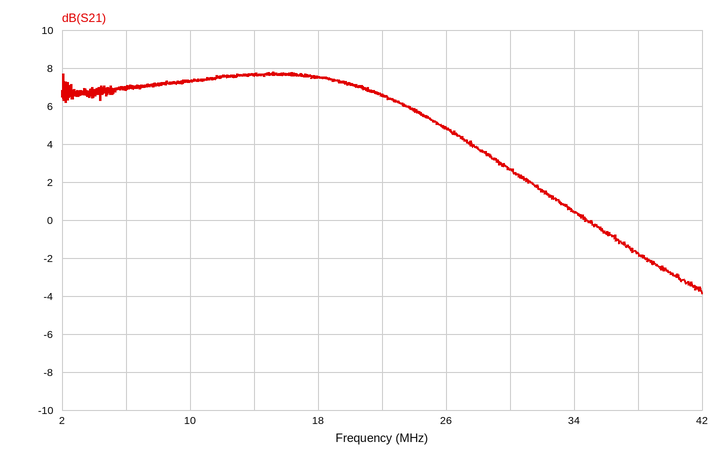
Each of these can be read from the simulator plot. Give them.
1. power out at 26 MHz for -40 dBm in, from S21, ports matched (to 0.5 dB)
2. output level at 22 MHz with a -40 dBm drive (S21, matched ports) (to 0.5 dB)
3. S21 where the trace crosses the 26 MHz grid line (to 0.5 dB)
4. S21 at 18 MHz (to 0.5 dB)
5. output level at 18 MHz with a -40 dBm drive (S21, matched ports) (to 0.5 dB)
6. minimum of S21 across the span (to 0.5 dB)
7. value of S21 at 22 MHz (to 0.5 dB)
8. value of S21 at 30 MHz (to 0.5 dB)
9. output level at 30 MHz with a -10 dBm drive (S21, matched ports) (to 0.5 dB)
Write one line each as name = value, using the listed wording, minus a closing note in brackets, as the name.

power out at 26 MHz for -40 dBm in, from S21, ports matched = -35.0 dBm
output level at 22 MHz with a -40 dBm drive (S21, matched ports) = -33.5 dBm
S21 where the trace crosses the 26 MHz grid line = 5.0 dB
S21 at 18 MHz = 7.5 dB
output level at 18 MHz with a -40 dBm drive (S21, matched ports) = -32.5 dBm
minimum of S21 across the span = -4.0 dB
value of S21 at 22 MHz = 6.5 dB
value of S21 at 30 MHz = 2.5 dB
output level at 30 MHz with a -10 dBm drive (S21, matched ports) = -7.5 dBm
